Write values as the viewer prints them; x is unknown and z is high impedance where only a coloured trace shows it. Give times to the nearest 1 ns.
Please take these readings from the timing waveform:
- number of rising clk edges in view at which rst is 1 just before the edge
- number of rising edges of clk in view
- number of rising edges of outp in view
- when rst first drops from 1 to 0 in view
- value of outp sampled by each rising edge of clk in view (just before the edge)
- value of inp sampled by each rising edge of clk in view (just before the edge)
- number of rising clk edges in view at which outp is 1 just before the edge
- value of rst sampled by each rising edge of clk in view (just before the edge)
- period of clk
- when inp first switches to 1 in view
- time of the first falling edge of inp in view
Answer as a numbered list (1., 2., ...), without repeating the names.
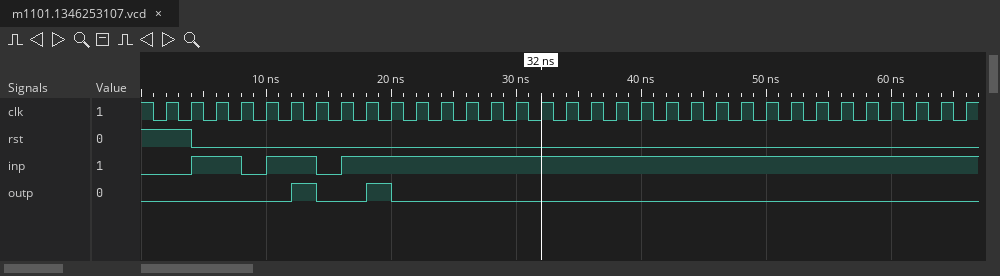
1. 2
2. 33
3. 2
4. 4 ns
5. 0 0 0 0 0 0 1 0 0 1 0 0 0 0 0 0 0 0 0 0 0 0 0 0 0 0 0 0 0 0 0 0 0
6. 0 0 1 1 0 1 1 0 1 1 1 1 1 1 1 1 1 1 1 1 1 1 1 1 1 1 1 1 1 1 1 1 1
7. 2
8. 1 1 0 0 0 0 0 0 0 0 0 0 0 0 0 0 0 0 0 0 0 0 0 0 0 0 0 0 0 0 0 0 0
9. 2 ns
10. 4 ns
11. 8 ns
